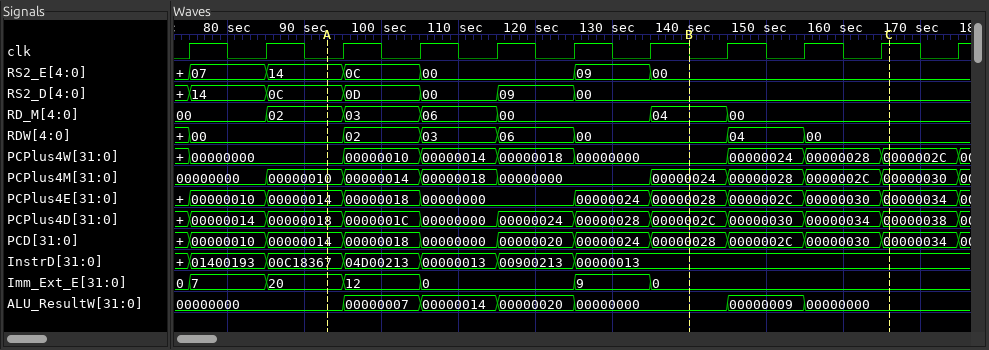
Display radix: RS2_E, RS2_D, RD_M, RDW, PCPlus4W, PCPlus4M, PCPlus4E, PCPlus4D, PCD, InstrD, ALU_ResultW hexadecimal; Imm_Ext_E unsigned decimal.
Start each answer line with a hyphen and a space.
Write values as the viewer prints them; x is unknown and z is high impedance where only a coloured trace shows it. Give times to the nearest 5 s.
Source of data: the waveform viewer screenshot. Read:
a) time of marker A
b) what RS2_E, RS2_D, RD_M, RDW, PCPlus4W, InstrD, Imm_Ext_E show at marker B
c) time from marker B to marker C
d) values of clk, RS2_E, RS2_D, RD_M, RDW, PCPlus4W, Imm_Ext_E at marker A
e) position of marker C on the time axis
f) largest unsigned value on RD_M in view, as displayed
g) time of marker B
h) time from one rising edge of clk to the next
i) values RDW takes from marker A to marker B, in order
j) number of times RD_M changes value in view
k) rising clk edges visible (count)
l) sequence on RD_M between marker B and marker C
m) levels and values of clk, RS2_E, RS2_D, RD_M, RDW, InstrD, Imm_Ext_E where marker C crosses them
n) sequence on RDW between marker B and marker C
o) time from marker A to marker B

- 95 s
- RS2_E=00, RS2_D=00, RD_M=04, RDW=00, PCPlus4W=00000000, InstrD=00000013, Imm_Ext_E=0
- 25 s
- clk=0, RS2_E=14, RS2_D=0C, RD_M=02, RDW=00, PCPlus4W=00000000, Imm_Ext_E=20
- 165 s
- 06
- 140 s
- 10 s
- 00, 02, 03, 06, 00
- 6
- 11
- 04, 00
- clk=1, RS2_E=00, RS2_D=00, RD_M=00, RDW=00, InstrD=00000013, Imm_Ext_E=0
- 00, 04, 00
- 45 s
